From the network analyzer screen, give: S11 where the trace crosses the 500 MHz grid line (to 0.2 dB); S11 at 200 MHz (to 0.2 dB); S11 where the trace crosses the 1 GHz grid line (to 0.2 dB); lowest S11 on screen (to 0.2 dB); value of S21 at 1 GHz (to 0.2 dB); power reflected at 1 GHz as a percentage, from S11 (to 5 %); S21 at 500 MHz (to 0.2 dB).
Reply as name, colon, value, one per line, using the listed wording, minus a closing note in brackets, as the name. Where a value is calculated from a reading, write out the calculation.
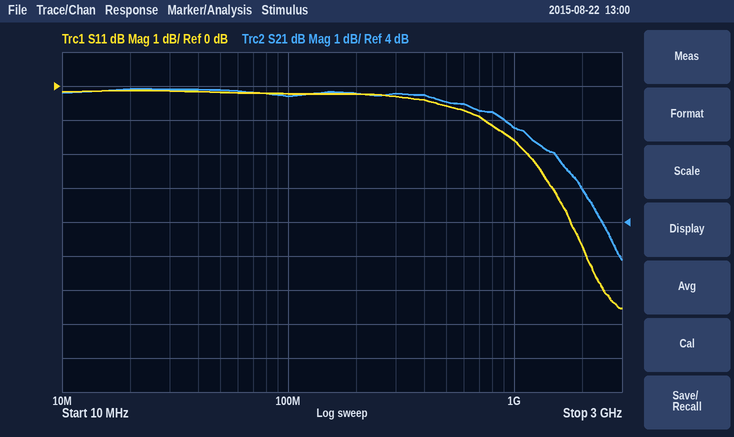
S11 where the trace crosses the 500 MHz grid line: -0.6 dB
S11 at 200 MHz: -0.2 dB
S11 where the trace crosses the 1 GHz grid line: -1.6 dB
lowest S11 on screen: -6.6 dB
value of S21 at 1 GHz: 6.8 dB
power reflected at 1 GHz as a percentage, from S11: 10^(-1.6/10) ≈ 69.2 %, so 70 % to the nearest 5 %
S21 at 500 MHz: 7.6 dB
